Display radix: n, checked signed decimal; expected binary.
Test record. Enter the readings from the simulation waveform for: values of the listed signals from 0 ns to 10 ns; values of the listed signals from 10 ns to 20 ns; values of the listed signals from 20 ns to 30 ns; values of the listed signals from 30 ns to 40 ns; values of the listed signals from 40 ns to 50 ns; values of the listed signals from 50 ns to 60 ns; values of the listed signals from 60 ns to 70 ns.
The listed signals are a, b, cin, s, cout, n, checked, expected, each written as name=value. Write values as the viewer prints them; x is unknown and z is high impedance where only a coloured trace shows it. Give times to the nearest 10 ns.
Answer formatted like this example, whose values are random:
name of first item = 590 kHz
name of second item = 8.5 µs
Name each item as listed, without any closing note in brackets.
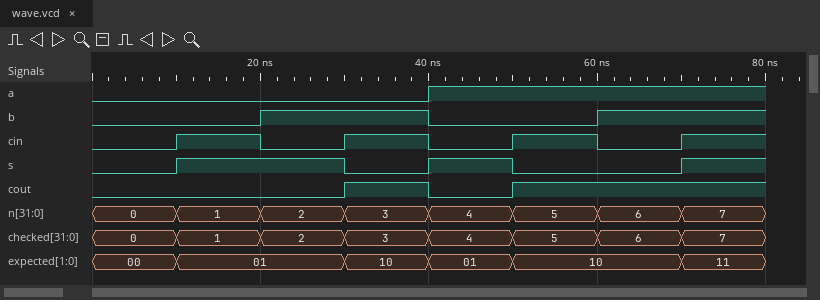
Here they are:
values of the listed signals from 0 ns to 10 ns = a=0, b=0, cin=0, s=0, cout=0, n=0, checked=0, expected=00
values of the listed signals from 10 ns to 20 ns = a=0, b=0, cin=1, s=1, cout=0, n=1, checked=1, expected=01
values of the listed signals from 20 ns to 30 ns = a=0, b=1, cin=0, s=1, cout=0, n=2, checked=2, expected=01
values of the listed signals from 30 ns to 40 ns = a=0, b=1, cin=1, s=0, cout=1, n=3, checked=3, expected=10
values of the listed signals from 40 ns to 50 ns = a=1, b=0, cin=0, s=1, cout=0, n=4, checked=4, expected=01
values of the listed signals from 50 ns to 60 ns = a=1, b=0, cin=1, s=0, cout=1, n=5, checked=5, expected=10
values of the listed signals from 60 ns to 70 ns = a=1, b=1, cin=0, s=0, cout=1, n=6, checked=6, expected=10
